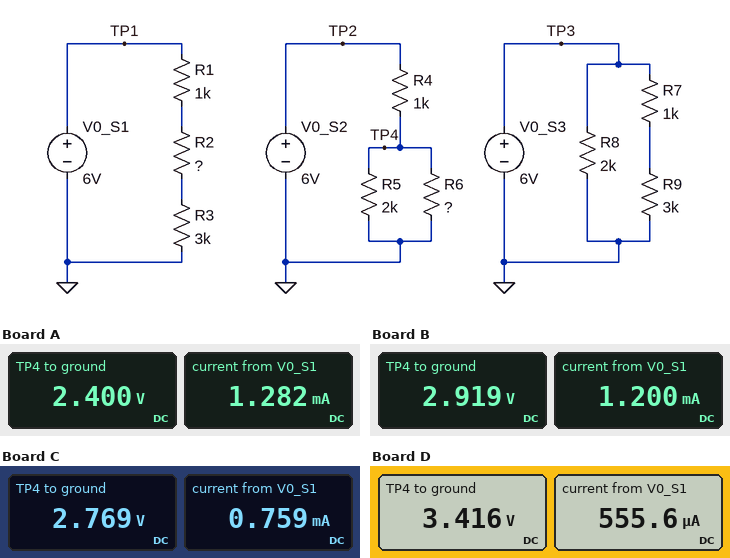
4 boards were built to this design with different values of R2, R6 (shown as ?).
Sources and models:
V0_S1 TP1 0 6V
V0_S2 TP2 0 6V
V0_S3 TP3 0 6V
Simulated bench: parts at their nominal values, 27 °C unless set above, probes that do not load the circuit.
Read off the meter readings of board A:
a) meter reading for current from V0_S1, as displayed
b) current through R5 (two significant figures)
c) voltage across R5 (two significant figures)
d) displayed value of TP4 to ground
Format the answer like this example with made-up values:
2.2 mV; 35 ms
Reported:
1.282 mA; 1.2 mA; 2.4 V; 2.400 V
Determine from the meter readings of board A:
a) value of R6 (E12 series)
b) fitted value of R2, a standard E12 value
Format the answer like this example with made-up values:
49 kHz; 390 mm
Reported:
1 kΩ; 680 Ω
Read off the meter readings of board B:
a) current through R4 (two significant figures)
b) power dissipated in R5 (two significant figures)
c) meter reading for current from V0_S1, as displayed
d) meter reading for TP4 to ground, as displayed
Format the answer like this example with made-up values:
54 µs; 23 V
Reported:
3.1 mA; 4.3 mW; 1.200 mA; 2.919 V
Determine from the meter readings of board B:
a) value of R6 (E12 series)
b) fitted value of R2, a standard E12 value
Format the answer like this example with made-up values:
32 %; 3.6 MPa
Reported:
1.8 kΩ; 1 kΩ
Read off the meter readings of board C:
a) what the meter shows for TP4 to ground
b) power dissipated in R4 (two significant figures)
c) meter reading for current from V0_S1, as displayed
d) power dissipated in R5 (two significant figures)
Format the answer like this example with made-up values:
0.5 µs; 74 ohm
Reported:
2.769 V; 10 mW; 0.759 mA; 3.8 mW
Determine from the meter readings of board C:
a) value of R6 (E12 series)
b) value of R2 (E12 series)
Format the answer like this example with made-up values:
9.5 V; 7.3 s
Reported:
1.5 kΩ; 3.9 kΩ
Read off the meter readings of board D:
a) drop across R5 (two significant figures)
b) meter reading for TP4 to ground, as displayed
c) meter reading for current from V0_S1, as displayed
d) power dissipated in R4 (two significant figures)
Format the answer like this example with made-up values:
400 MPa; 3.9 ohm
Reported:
3.4 V; 3.416 V; 555.6 µA; 6.7 mW
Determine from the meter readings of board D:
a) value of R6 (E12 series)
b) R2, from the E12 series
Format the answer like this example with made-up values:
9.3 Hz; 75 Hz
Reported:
3.9 kΩ; 6.8 kΩ
